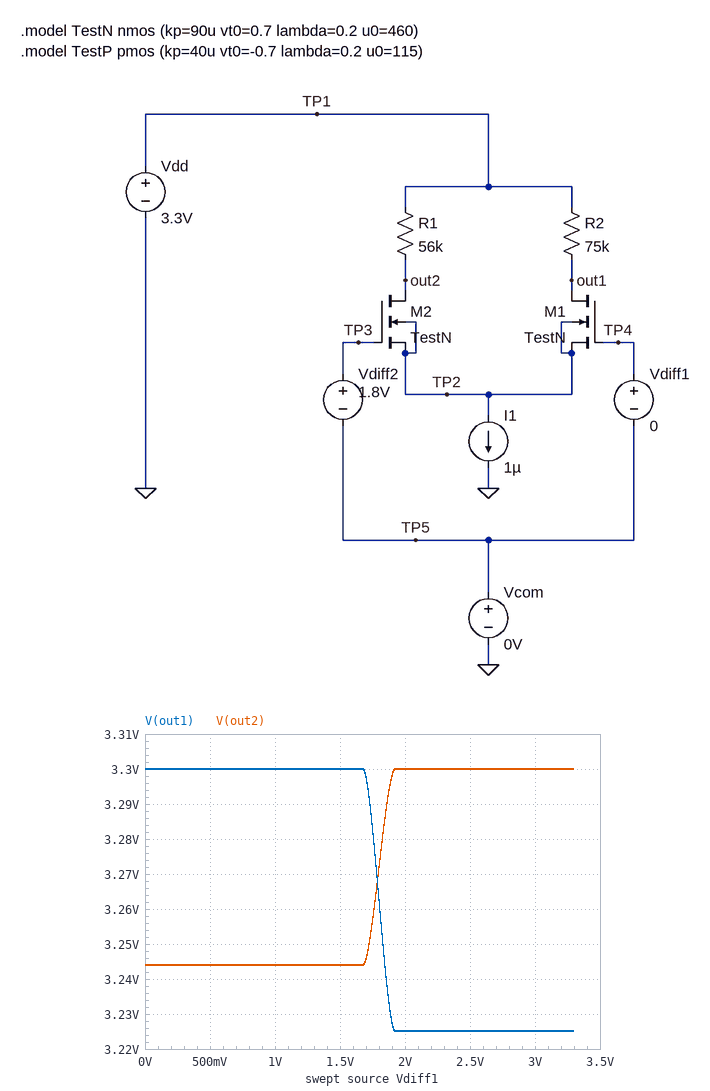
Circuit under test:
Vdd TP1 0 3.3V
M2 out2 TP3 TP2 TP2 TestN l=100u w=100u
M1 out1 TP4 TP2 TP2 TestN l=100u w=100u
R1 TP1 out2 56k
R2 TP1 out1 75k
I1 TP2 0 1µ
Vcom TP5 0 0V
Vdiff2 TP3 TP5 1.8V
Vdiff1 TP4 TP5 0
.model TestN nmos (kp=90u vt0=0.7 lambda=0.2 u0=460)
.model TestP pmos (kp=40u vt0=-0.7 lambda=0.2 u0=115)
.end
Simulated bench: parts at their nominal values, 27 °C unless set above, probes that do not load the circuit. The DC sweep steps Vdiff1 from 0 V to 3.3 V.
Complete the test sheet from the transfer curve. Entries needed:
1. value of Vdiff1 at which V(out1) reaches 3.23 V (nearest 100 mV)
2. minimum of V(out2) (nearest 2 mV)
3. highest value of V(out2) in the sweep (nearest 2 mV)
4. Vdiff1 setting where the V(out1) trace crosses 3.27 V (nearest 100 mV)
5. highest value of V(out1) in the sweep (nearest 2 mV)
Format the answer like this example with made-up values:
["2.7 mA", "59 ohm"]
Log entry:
["1.9 V", "3.244 V", "3.300 V", "1.8 V", "3.300 V"]
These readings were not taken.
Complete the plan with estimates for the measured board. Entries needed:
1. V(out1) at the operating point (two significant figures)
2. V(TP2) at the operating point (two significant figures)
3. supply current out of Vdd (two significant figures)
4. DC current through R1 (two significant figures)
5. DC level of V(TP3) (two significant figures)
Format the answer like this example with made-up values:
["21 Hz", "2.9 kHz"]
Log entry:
["3.3 V", "980 mV", "1.0 µA", "1.0 µA", "1.8 V"]
